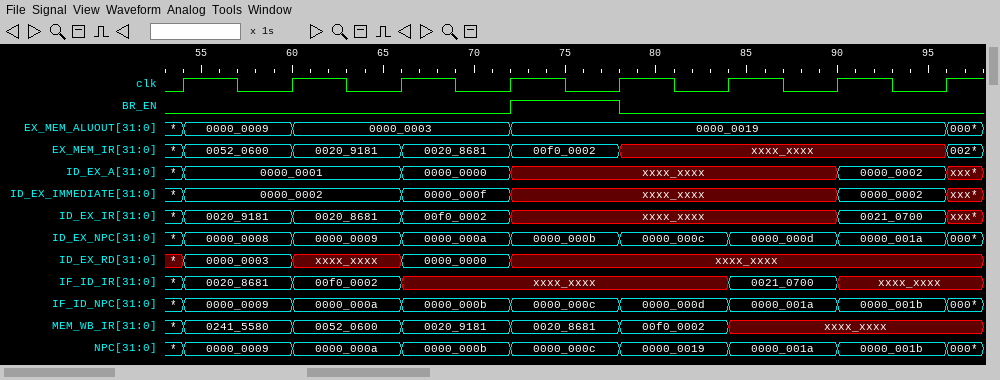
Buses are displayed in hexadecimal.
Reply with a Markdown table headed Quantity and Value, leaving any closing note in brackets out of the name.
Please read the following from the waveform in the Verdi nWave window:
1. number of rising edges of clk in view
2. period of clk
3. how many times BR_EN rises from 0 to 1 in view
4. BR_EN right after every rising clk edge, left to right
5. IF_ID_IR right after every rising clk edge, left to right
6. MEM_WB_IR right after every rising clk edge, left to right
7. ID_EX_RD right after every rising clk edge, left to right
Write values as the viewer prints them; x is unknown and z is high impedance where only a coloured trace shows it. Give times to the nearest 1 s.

| Quantity | Value |
|---|---|
| number of rising edges of clk in view | 8 |
| period of clk | 6 s |
| how many times BR_EN rises from 0 to 1 in view | 1 |
| BR_EN right after every rising clk edge, left to right | 0 0 0 1 0 0 0 0 |
| IF_ID_IR right after every rising clk edge, left to right | 0020_8681, 00f0_0002, xxxx_xxxx, xxxx_xxxx, xxxx_xxxx, 0021_0700, xxxx_xxxx, xxxx_xxxx |
| MEM_WB_IR right after every rising clk edge, left to right | 0241_5580, 0052_0600, 0020_9181, 0020_8681, 00f0_0002, xxxx_xxxx, xxxx_xxxx, xxxx_xxxx |
| ID_EX_RD right after every rising clk edge, left to right | 0000_0003, xxxx_xxxx, 0000_0000, xxxx_xxxx, xxxx_xxxx, xxxx_xxxx, xxxx_xxxx, xxxx_xxxx |
